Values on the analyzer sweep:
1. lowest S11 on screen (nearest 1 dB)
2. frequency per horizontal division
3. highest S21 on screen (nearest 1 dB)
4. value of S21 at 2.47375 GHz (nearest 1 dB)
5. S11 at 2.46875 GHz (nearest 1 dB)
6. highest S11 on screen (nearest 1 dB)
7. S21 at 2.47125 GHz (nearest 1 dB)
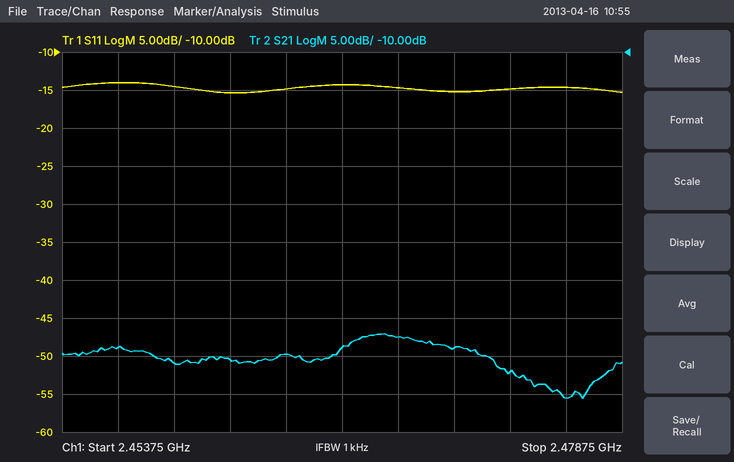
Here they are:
-15 dB
2.5 MHz
-47 dB
-52 dB
-15 dB
-14 dB
-49 dB
